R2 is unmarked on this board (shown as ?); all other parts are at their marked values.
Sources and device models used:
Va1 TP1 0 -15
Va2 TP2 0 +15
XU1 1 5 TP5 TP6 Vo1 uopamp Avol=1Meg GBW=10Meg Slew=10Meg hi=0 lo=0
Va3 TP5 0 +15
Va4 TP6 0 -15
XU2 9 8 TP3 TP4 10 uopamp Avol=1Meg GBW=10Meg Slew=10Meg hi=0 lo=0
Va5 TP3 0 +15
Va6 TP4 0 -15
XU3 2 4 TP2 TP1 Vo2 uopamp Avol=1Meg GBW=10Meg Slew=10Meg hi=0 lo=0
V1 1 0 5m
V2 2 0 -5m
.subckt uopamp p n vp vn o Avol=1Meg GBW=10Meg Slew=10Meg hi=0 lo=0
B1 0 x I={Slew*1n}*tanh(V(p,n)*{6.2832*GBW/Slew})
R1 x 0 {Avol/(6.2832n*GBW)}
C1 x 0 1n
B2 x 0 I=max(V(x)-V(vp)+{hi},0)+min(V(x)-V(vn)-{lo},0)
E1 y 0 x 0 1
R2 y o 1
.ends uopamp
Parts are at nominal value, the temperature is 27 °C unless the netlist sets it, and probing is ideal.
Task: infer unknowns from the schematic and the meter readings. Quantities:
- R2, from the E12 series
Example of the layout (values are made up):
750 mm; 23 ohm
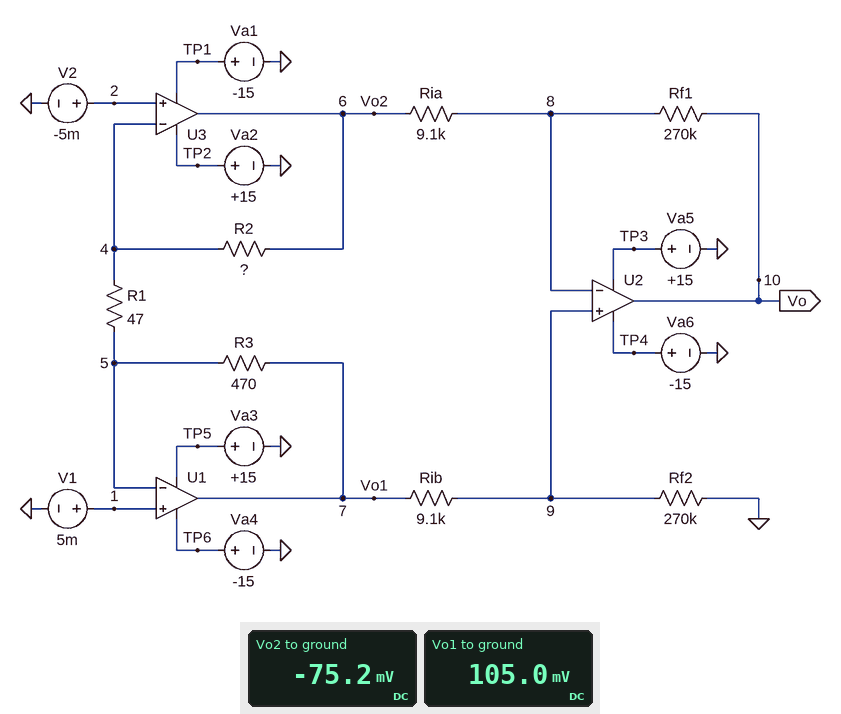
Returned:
330 Ω
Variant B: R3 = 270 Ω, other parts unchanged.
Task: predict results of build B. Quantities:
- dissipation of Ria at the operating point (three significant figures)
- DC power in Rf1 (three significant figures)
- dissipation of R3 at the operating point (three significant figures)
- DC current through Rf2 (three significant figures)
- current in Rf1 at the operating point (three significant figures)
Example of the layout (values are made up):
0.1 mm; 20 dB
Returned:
2.02 µW; 60.0 µW; 12.2 µW; 224 nA; 14.9 µA
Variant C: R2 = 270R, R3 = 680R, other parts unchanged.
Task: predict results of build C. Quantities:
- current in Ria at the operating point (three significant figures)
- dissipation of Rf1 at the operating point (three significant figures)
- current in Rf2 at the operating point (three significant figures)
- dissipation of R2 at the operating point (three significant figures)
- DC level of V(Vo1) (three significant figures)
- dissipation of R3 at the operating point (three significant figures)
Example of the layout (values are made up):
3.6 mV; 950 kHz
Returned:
22.8 µA; 140 µW; 536 nA; 12.2 µW; 150 mV; 30.8 µW
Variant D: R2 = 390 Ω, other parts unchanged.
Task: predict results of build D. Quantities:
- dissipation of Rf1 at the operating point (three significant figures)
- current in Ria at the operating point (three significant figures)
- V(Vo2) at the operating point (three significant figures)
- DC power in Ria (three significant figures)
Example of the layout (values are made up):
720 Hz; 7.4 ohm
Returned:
117 µW; 20.8 µA; -88.0 mV; 3.95 µW
